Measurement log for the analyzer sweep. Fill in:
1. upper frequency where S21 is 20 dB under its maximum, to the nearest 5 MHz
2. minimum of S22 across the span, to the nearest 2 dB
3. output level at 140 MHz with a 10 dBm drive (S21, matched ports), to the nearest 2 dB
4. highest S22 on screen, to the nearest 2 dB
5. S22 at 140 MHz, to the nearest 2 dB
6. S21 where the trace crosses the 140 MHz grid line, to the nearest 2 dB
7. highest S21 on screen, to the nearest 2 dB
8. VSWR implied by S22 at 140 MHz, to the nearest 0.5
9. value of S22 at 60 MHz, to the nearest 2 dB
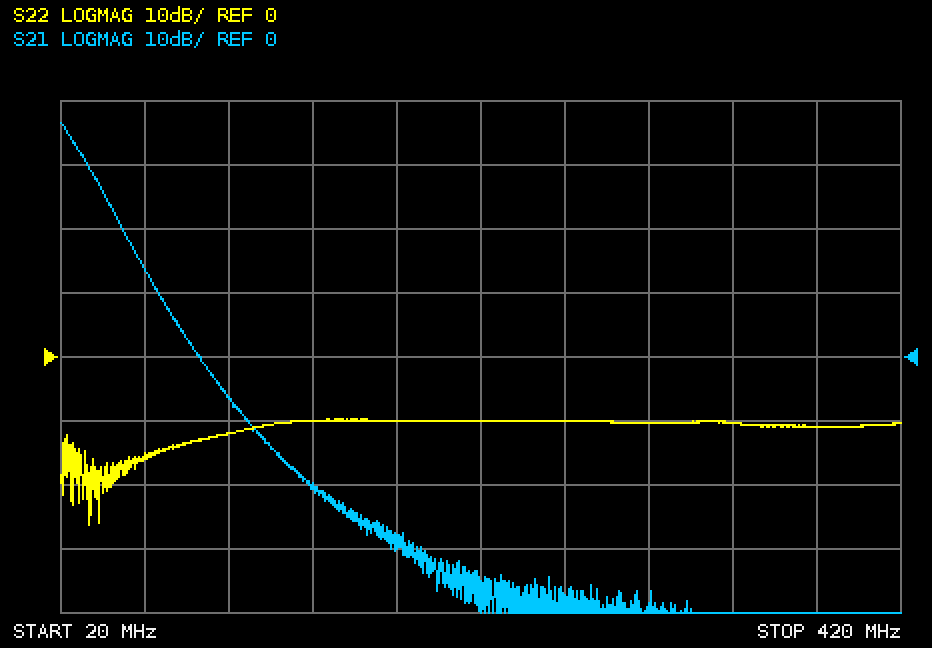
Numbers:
55 MHz
-26 dB
-10 dBm
-10 dB
-10 dB
-20 dB
36 dB
2.0
-16 dB
